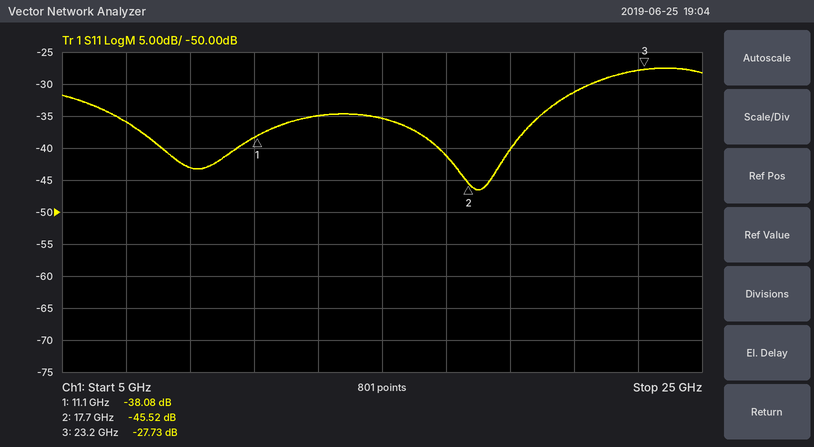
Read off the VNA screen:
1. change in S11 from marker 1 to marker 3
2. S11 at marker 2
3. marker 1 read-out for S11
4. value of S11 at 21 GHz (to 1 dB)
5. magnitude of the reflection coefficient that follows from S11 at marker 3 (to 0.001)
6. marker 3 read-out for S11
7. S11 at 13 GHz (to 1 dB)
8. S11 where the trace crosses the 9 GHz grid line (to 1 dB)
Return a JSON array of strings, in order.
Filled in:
["10.35 dB", "-45.52 dB", "-38.08 dB", "-31 dB", "0.041", "-27.73 dB", "-35 dB", "-43 dB"]
